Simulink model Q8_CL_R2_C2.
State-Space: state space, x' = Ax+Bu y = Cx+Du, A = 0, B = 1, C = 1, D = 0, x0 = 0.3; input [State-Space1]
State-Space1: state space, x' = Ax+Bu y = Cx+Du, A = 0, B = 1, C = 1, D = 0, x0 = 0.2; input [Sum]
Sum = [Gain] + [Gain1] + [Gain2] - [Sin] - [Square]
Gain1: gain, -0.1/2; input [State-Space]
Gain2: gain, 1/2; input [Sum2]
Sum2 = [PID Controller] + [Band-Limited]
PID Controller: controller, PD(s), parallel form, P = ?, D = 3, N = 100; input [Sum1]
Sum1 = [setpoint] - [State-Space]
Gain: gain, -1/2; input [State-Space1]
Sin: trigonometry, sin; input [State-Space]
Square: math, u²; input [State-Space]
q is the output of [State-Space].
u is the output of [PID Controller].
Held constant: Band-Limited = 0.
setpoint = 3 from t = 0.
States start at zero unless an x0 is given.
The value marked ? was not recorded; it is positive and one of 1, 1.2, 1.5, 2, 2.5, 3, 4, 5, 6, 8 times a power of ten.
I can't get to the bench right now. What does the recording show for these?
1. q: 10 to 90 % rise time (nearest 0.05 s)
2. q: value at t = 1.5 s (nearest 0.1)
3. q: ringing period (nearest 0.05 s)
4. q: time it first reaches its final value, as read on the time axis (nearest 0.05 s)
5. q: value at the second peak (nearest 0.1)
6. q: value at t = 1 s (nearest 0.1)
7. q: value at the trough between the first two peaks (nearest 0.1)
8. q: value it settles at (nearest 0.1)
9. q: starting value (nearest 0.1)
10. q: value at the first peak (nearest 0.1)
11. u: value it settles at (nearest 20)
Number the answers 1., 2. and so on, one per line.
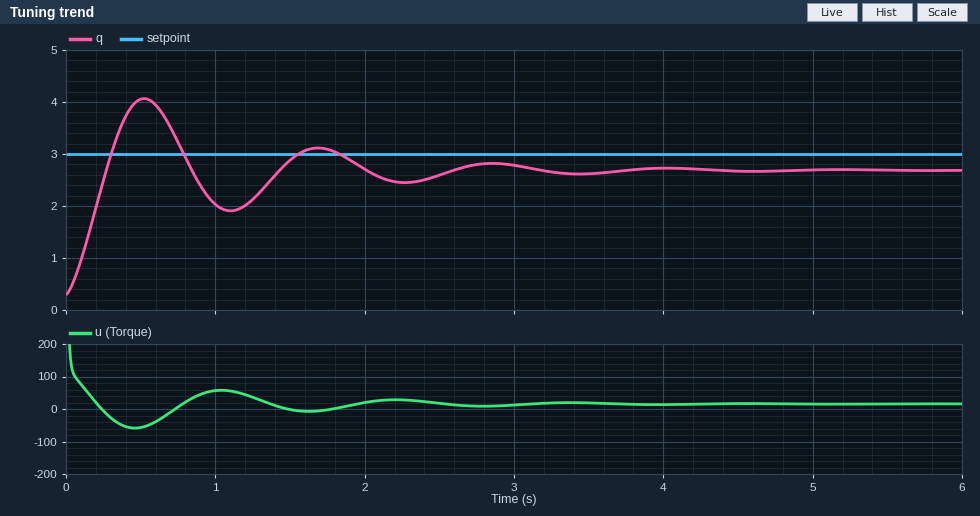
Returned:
1. 0.20 s
2. 2.9
3. 1.15 s
4. 0.25 s
5. 3.1
6. 2.0
7. 1.9
8. 2.7
9. 0.3
10. 4.1
11. 20
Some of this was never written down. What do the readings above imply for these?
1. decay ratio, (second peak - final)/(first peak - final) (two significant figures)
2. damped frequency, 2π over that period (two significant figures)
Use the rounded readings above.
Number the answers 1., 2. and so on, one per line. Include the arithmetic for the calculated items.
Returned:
1. (3.1 - 2.7) / (4.1 - 2.7) = 0.29
2. 2π / 1.15 = 5.5 rad/s
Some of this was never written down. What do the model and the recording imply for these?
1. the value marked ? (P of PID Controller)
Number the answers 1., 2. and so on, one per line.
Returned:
1. 50
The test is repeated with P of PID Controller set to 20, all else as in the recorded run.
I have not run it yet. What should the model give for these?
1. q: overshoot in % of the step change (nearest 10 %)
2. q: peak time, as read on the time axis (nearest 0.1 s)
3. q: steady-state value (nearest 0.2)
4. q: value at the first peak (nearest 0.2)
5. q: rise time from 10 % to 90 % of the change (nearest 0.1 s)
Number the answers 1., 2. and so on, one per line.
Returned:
1. 50 %
2. 0.7 s
3. 2.4
4. 3.4
5. 0.3 s
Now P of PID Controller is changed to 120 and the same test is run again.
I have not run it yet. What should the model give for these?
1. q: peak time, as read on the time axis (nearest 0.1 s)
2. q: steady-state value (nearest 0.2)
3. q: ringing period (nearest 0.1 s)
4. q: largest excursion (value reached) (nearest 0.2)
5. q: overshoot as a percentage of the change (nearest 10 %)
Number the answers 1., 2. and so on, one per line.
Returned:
1. 0.4 s
2. 2.8
3. 0.8 s
4. 4.6
5. 70 %
